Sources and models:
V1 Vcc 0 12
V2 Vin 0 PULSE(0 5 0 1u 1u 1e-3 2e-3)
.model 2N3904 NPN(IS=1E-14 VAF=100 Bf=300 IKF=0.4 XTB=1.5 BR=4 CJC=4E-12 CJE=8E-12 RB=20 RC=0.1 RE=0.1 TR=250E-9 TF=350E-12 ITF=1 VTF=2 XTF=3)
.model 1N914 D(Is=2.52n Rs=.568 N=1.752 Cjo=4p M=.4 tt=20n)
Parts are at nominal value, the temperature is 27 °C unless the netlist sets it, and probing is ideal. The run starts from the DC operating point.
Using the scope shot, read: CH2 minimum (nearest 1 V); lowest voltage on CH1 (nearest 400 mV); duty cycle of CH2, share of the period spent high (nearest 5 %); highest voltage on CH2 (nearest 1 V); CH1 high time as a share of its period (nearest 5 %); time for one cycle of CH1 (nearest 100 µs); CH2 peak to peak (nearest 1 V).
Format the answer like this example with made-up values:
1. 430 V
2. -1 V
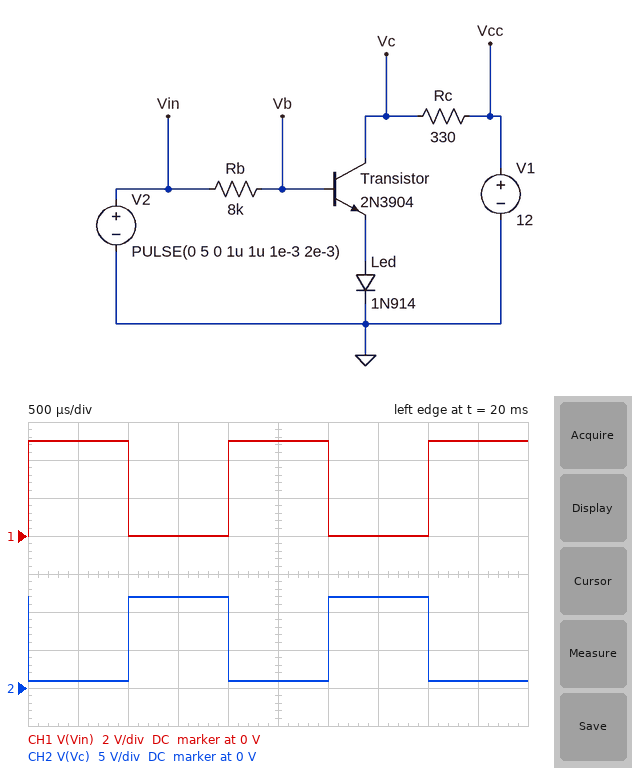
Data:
1. 1 V
2. 0 V
3. 50 %
4. 12 V
5. 50 %
6. 2.0 ms
7. 11 V
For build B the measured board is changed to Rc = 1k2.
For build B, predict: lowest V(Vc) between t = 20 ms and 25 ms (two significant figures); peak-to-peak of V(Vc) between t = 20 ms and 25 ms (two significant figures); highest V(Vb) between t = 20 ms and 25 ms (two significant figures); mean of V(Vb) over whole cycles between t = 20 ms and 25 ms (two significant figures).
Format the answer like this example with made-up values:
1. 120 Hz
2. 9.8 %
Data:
1. 750 mV
2. 11 V
3. 1.4 V
4. 710 mV
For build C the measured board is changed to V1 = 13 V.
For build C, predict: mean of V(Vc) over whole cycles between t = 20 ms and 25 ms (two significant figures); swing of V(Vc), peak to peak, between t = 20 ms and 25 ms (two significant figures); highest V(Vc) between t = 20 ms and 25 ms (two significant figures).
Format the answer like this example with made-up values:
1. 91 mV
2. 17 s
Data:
1. 6.9 V
2. 12 V
3. 13 V
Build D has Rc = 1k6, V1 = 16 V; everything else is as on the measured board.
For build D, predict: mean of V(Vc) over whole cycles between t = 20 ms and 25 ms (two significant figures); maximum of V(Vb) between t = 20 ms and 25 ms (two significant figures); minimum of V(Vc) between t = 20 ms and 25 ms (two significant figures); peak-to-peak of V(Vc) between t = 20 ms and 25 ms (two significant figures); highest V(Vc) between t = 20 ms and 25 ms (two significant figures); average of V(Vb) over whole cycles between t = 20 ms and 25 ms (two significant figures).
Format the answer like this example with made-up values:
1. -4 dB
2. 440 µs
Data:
1. 8.4 V
2. 1.4 V
3. 750 mV
4. 15 V
5. 16 V
6. 710 mV
